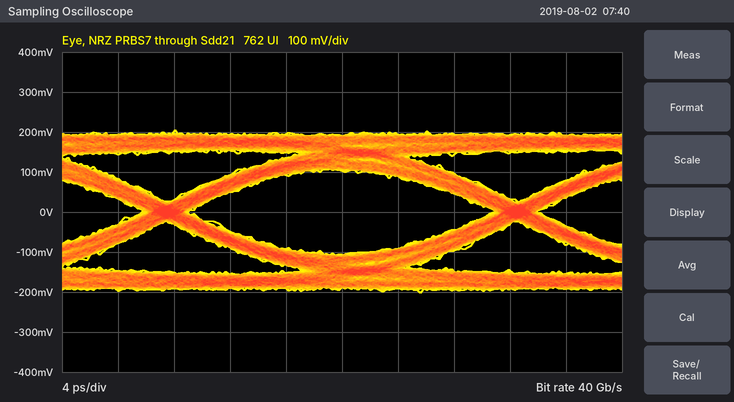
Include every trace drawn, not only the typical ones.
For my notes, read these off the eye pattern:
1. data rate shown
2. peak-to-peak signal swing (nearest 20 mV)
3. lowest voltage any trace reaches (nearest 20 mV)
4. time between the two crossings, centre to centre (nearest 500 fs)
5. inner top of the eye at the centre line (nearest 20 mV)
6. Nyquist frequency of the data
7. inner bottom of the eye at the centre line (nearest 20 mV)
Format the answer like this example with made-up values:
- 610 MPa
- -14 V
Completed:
- 40 Gb/s
- 400 mV
- -200 mV
- 25.0 ps
- 100 mV
- 20 GHz
- -100 mV
